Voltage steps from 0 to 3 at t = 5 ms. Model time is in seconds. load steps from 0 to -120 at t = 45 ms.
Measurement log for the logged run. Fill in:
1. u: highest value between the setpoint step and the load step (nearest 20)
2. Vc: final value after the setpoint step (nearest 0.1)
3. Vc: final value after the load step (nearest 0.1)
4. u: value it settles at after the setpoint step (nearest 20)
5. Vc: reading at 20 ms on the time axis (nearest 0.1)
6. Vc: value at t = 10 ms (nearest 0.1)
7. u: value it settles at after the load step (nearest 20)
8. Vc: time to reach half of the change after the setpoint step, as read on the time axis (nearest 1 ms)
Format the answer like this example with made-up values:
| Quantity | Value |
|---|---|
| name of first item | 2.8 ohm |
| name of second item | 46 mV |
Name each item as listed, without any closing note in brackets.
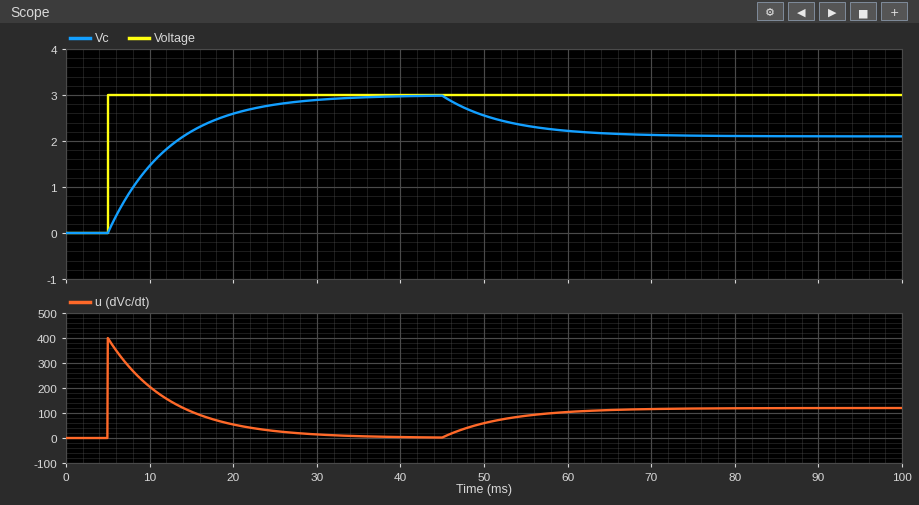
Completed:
| Quantity | Value |
|---|---|
| u: highest value between the setpoint step and the load step | 400 |
| Vc: final value after the setpoint step | 3.0 |
| Vc: final value after the load step | 2.1 |
| u: value it settles at after the setpoint step | 0 |
| Vc: reading at 20 ms on the time axis | 2.6 |
| Vc: value at t = 10 ms | 1.5 |
| u: value it settles at after the load step | 120 |
| Vc: time to reach half of the change after the setpoint step, as read on the time axis | 10 ms |
